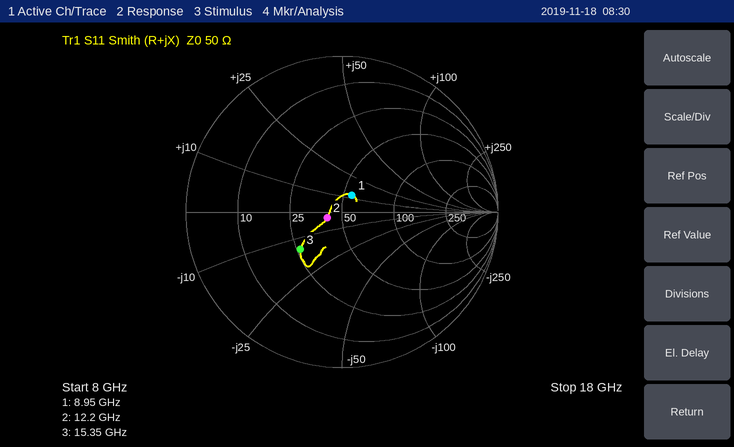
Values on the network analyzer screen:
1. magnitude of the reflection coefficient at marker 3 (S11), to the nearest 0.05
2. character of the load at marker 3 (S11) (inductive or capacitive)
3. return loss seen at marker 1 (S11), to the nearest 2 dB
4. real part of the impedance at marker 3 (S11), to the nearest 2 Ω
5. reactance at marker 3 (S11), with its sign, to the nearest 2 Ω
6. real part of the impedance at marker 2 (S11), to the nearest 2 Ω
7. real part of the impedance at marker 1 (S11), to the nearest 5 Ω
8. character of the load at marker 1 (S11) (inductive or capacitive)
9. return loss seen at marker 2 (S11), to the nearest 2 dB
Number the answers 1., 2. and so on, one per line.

1. 0.35
2. capacitive
3. 18 dB
4. 26 Ω
5. -14 Ω
6. 42 Ω
7. 55 Ω
8. inductive
9. 20 dB
